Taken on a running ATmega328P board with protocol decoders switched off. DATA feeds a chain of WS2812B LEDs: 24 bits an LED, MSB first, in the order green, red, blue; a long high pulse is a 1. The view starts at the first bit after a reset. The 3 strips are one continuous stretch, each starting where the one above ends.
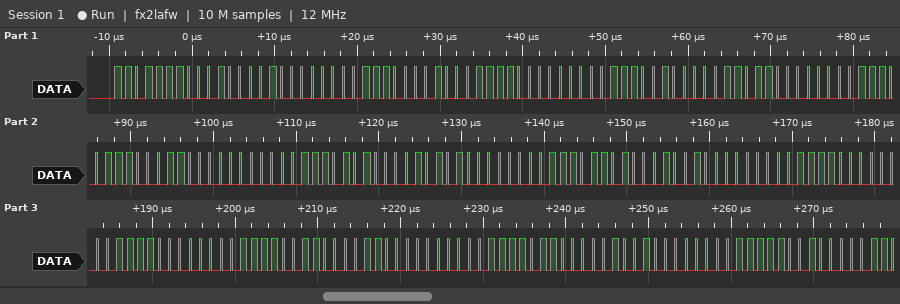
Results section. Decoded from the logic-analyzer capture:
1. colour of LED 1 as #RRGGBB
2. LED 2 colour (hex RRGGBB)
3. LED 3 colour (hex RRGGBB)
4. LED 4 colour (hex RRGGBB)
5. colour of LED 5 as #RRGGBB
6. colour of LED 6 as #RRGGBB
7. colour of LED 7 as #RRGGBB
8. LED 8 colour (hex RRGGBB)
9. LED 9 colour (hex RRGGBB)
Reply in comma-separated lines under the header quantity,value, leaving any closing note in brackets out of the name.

quantity,value
colour of LED 1 as #RRGGBB,#21DE00
LED 2 colour,#1EE100
LED 3 colour,#1BE400
LED 4 colour,#18E700
colour of LED 5 as #RRGGBB,#15EA00
colour of LED 6 as #RRGGBB,#12ED00
colour of LED 7 as #RRGGBB,#0FF000
LED 8 colour,#0CF300
LED 9 colour,#09F600
